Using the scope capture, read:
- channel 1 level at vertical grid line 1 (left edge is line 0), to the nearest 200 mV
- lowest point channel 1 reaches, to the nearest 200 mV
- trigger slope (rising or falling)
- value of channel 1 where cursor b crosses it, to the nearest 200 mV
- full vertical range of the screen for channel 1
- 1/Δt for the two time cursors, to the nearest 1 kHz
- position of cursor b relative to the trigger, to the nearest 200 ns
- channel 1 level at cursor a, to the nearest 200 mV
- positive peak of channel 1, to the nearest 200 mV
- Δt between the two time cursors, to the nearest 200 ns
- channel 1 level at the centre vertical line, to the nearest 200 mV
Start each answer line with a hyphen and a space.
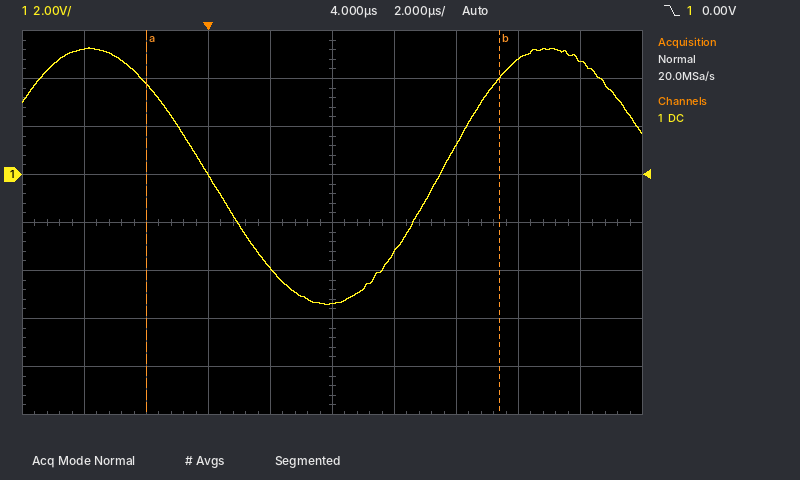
- 5.2 V
- -5.4 V
- falling
- 4.0 V
- 16 V
- 88 kHz
- +9.4 µs
- 3.8 V
- 5.2 V
- 11.4 µs
- -5.4 V
